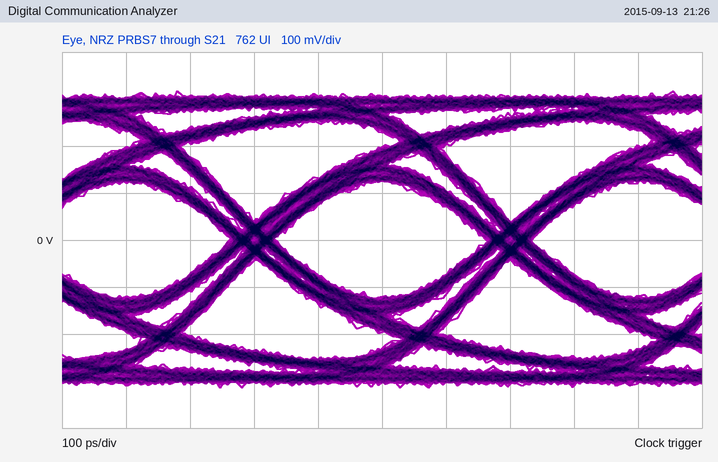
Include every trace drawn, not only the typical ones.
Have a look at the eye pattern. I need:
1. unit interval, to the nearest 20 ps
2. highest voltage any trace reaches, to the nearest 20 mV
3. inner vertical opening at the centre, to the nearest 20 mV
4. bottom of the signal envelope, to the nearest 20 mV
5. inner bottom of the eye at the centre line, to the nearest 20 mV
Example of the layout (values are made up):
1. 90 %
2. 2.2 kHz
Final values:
1. 400 ps
2. 320 mV
3. 240 mV
4. -320 mV
5. -120 mV
